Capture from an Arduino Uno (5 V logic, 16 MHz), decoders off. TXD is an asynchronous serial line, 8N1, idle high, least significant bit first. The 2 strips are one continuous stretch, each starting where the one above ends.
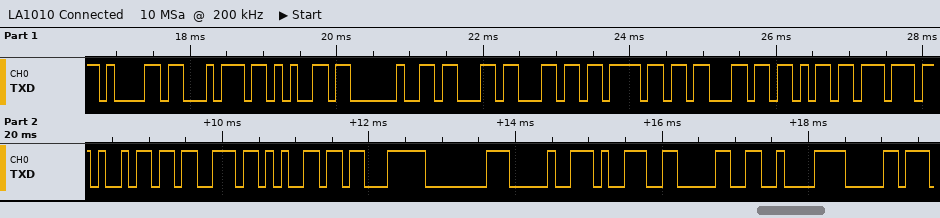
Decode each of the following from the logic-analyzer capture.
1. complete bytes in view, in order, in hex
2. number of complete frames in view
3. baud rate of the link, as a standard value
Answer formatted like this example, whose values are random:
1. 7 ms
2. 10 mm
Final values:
1. 0x61 0x74 0x65 0x20 0x63 0x6C 0x6F 0x63 0x6B 0x77 0x69 0x73 0x65 0xE3 0x80 0x90 0x39 0x30 0xC2 0xB0
2. 20
3. 9600 baud
